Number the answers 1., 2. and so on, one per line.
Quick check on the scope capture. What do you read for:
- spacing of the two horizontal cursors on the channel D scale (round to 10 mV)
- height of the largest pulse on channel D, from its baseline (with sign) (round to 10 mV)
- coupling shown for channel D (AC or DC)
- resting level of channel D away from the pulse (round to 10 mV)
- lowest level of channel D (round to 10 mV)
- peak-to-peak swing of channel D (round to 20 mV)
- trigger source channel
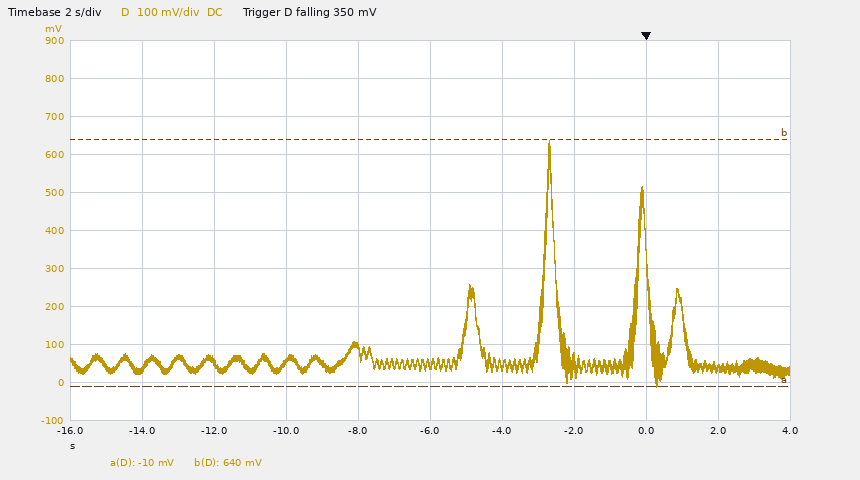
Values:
1. 650 mV
2. +590 mV
3. DC
4. 50 mV
5. -10 mV
6. 640 mV
7. channel D
